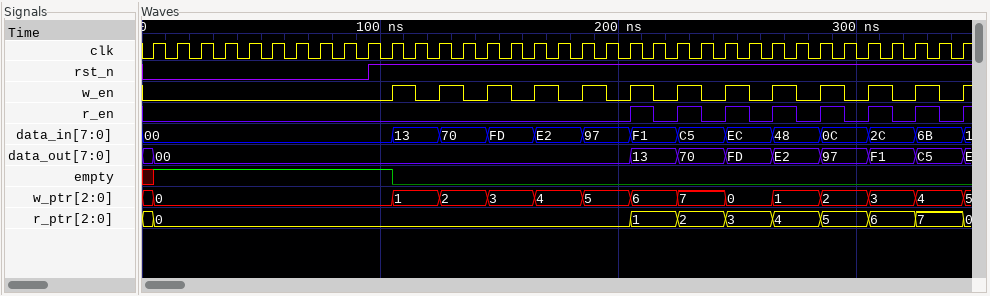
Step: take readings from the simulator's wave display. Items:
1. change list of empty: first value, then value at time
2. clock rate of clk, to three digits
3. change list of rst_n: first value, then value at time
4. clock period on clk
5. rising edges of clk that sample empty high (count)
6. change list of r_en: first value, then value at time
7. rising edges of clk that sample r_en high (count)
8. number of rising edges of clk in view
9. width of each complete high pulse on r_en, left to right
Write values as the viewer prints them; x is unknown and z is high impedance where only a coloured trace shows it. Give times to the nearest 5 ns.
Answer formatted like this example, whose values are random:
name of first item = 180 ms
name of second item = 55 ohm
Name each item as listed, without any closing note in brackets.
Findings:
change list of empty: first value, then value at time = x, 1 at 5 ns, 0 at 105 ns
clock rate of clk, to three digits = 100 MHz
change list of rst_n: first value, then value at time = 0, 1 at 95 ns
clock period on clk = 10 ns
rising edges of clk that sample empty high = 10
change list of r_en: first value, then value at time = 0, 1 at 205 ns, 0 at 215 ns, 1 at 225 ns, 0 at 235 ns, 1 at 245 ns, 0 at 255 ns, 1 at 265 ns, 0 at 275 ns, 1 at 285 ns, 0 at 295 ns, 1 at 305 ns, 0 at 315 ns, 1 at 325 ns, 0 at 335 ns, 1 at 345 ns
rising edges of clk that sample r_en high = 7
number of rising edges of clk in view = 35
width of each complete high pulse on r_en, left to right = 10 ns, 10 ns, 10 ns, 10 ns, 10 ns, 10 ns, 10 ns
